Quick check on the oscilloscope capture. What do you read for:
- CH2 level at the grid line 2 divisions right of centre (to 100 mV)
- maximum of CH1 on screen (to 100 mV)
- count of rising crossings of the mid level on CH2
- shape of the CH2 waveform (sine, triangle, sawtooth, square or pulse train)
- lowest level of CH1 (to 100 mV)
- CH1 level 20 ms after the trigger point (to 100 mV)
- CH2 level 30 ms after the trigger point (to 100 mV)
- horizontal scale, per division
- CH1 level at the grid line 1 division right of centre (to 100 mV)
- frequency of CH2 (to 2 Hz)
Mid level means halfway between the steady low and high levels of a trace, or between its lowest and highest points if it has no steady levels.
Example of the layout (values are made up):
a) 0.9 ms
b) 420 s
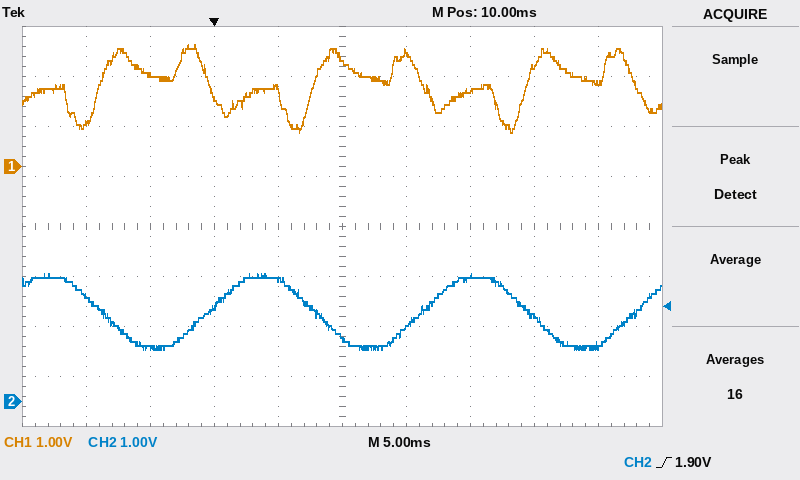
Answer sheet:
a) 2.5 V
b) 2.4 V
c) 3
d) sine
e) 700 mV
f) 1.5 V
g) 1.1 V
h) 5 ms
i) 2.3 V
j) 60 Hz
